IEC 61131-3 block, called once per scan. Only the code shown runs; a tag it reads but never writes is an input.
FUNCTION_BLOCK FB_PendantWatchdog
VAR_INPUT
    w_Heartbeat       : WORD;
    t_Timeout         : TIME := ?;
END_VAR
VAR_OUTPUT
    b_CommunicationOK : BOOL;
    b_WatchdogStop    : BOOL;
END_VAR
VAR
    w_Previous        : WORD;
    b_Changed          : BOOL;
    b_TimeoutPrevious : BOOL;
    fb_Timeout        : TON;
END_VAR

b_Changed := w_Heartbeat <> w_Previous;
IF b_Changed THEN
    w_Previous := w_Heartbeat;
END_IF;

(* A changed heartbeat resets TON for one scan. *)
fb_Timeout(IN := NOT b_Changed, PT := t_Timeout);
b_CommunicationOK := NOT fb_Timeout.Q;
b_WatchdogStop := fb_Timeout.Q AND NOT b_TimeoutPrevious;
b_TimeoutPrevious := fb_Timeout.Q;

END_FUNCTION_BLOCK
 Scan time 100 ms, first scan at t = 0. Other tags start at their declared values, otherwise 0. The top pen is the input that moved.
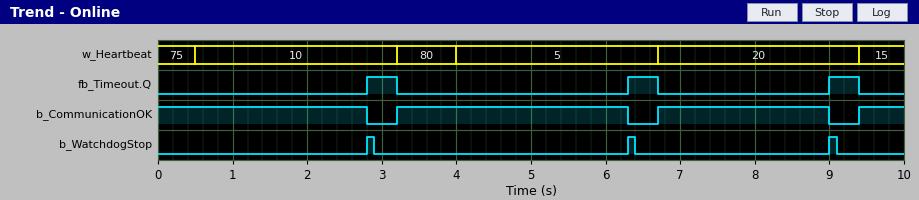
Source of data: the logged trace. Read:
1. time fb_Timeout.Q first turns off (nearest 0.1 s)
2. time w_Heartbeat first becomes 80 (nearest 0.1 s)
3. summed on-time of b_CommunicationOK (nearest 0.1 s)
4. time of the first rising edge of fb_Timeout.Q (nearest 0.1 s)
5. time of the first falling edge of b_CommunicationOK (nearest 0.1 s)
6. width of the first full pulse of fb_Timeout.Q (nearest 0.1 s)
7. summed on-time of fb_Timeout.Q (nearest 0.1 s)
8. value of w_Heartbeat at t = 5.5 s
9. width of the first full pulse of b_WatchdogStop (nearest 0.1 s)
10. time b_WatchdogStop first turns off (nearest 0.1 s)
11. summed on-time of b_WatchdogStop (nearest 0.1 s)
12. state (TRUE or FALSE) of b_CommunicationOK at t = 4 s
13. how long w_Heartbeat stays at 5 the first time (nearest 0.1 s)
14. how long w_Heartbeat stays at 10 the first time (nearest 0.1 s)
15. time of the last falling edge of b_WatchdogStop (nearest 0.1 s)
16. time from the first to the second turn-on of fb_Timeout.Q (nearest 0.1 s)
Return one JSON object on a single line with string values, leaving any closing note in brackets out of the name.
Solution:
{"time fb_Timeout.Q first turns off": "3.2 s", "time w_Heartbeat first becomes 80": "3.2 s", "summed on-time of b_CommunicationOK": "8.8 s", "time of the first rising edge of fb_Timeout.Q": "2.8 s", "time of the first falling edge of b_CommunicationOK": "2.8 s", "width of the first full pulse of fb_Timeout.Q": "0.4 s", "summed on-time of fb_Timeout.Q": "1.2 s", "value of w_Heartbeat at t = 5.5 s": "5", "width of the first full pulse of b_WatchdogStop": "0.1 s", "time b_WatchdogStop first turns off": "2.9 s", "summed on-time of b_WatchdogStop": "0.3 s", "state (TRUE or FALSE) of b_CommunicationOK at t = 4 s": "TRUE", "how long w_Heartbeat stays at 5 the first time": "2.7 s", "how long w_Heartbeat stays at 10 the first time": "2.7 s", "time of the last falling edge of b_WatchdogStop": "9.1 s", "time from the first to the second turn-on of fb_Timeout.Q": "3.5 s"}
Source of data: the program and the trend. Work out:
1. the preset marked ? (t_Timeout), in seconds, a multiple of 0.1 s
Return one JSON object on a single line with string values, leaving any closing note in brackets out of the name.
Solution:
{"the preset marked ? (t_Timeout), in seconds, a multiple of 0.1 s": "2.2 s"}
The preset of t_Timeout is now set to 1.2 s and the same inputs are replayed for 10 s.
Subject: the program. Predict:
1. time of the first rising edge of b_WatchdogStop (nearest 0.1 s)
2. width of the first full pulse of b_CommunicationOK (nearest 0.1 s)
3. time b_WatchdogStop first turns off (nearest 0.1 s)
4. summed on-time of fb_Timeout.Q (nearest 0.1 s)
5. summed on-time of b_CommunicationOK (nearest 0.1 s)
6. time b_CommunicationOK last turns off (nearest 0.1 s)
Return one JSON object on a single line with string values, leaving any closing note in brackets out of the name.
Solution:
{"time of the first rising edge of b_WatchdogStop": "1.8 s", "width of the first full pulse of b_CommunicationOK": "2.1 s", "time b_WatchdogStop first turns off": "1.9 s", "summed on-time of fb_Timeout.Q": "4.2 s", "summed on-time of b_CommunicationOK": "5.8 s", "time b_CommunicationOK last turns off": "8.0 s"}
